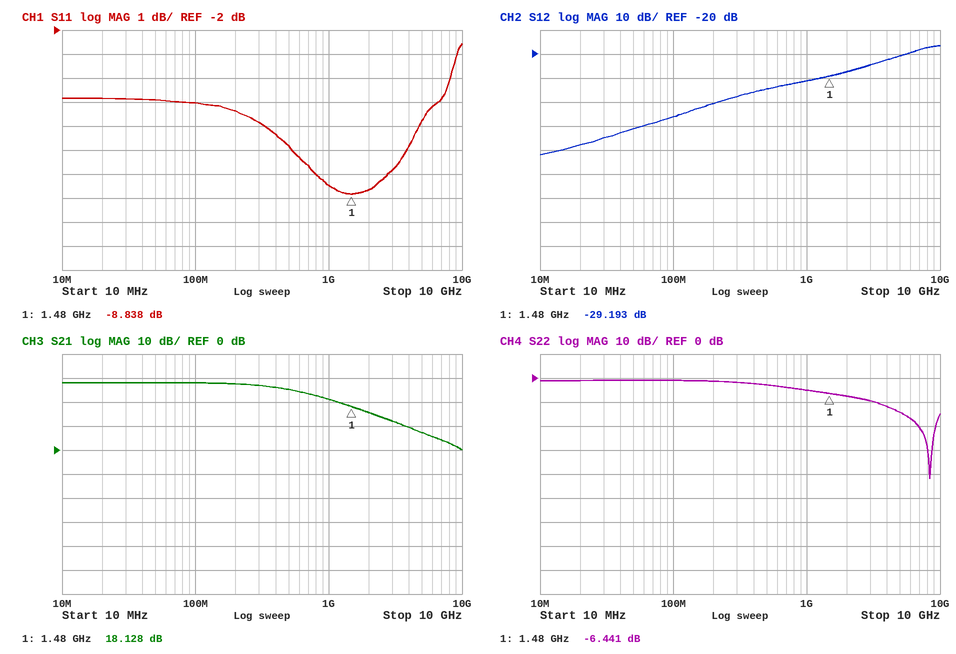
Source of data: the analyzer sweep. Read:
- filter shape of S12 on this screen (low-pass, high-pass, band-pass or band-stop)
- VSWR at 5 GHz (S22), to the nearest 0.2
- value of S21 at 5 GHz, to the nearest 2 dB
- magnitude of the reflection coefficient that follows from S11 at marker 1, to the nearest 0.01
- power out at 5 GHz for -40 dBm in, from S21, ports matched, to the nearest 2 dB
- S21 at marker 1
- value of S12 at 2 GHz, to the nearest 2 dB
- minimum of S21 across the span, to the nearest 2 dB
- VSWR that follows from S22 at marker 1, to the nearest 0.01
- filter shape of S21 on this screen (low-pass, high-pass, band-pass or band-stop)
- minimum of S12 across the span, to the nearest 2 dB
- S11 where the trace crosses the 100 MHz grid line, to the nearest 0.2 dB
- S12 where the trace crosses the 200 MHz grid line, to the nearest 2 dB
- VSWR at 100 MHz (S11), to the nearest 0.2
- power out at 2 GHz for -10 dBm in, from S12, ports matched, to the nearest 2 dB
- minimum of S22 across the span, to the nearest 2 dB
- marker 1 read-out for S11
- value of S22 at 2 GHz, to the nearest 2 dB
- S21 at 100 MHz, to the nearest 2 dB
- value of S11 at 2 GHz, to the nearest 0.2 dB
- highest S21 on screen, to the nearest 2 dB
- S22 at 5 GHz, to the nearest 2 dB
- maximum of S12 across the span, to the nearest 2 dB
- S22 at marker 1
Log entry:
high-pass
1.4
8 dB
0.36
-32 dBm
18.128 dB
-28 dB
0 dB
2.82
low-pass
-62 dB
-5.0 dB
-40 dB
3.6
-38 dBm
-42 dB
-8.838 dB
-8 dB
28 dB
-8.6 dB
28 dB
-14 dB
-16 dB
-6.441 dB
